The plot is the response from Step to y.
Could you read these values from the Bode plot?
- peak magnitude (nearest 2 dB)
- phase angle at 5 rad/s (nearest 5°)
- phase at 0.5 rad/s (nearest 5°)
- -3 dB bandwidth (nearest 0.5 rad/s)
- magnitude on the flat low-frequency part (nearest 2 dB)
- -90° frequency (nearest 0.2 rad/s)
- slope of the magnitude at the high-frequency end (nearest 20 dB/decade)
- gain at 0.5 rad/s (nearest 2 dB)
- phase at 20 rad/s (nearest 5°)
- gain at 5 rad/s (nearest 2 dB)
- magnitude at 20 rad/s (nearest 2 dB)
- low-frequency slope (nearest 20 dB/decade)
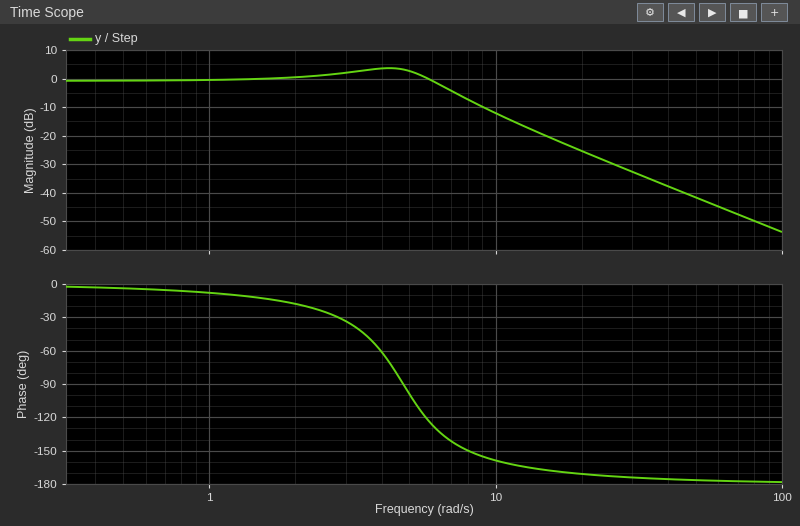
4 dB
-100°
-5°
7.0 rad/s
0 dB
4.8 rad/s
-40 dB/decade
0 dB
-170°
2 dB
-26 dB
0 dB/decade
